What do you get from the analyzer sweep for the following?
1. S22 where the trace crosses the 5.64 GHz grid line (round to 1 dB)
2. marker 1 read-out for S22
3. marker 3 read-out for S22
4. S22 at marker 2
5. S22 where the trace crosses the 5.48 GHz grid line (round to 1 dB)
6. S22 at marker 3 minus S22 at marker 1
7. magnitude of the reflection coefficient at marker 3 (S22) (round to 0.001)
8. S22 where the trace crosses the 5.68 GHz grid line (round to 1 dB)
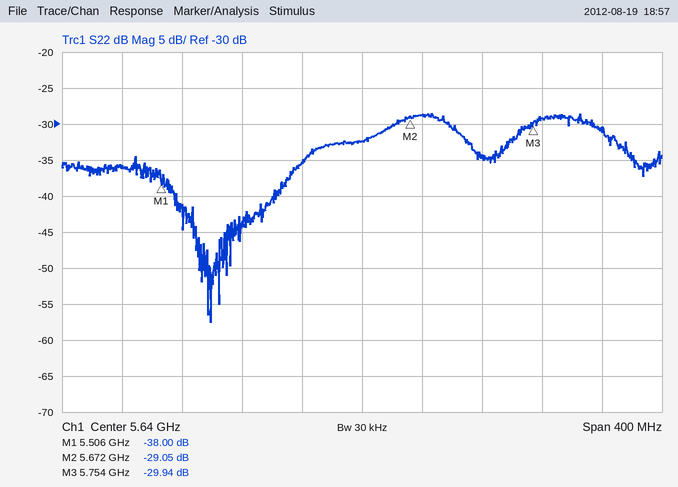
-32 dB
-38.00 dB
-29.94 dB
-29.05 dB
-36 dB
8.06 dB
0.032
-29 dB
